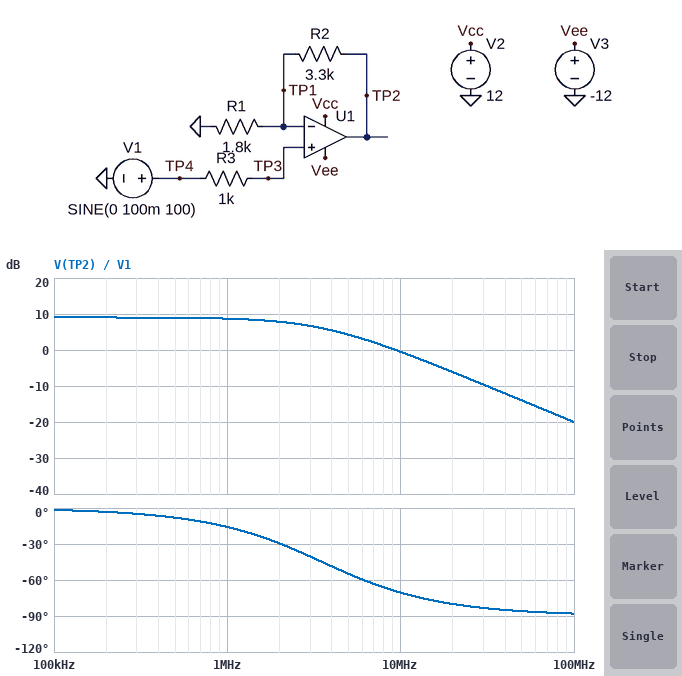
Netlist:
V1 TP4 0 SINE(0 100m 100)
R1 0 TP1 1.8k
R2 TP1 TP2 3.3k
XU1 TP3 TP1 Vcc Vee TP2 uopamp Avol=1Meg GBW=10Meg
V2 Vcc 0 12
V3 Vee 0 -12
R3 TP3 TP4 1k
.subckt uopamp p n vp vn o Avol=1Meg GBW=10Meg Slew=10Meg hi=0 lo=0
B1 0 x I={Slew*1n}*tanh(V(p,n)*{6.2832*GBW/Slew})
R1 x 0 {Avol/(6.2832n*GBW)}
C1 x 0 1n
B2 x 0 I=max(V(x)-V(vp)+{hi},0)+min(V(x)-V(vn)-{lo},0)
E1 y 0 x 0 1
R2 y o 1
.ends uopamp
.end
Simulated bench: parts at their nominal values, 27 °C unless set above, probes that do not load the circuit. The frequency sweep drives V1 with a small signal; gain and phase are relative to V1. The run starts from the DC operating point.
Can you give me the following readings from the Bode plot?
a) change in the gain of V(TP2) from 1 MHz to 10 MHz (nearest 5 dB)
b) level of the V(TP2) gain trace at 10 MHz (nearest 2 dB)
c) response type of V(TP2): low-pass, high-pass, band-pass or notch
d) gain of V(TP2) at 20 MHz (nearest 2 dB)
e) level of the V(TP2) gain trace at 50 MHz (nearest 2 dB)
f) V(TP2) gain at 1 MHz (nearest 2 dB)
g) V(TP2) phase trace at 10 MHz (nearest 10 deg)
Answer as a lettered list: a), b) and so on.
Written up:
a) -10 dB
b) 0 dB
c) low-pass
d) -6 dB
e) -14 dB
f) 8 dB
g) -70 deg
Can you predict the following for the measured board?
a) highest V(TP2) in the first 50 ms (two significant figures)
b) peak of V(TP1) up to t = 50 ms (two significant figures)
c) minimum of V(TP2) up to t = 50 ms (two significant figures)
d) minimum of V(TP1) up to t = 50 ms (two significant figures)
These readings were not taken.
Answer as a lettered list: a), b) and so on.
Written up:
a) 280 mV
b) 100 mV
c) -280 mV
d) -100 mV
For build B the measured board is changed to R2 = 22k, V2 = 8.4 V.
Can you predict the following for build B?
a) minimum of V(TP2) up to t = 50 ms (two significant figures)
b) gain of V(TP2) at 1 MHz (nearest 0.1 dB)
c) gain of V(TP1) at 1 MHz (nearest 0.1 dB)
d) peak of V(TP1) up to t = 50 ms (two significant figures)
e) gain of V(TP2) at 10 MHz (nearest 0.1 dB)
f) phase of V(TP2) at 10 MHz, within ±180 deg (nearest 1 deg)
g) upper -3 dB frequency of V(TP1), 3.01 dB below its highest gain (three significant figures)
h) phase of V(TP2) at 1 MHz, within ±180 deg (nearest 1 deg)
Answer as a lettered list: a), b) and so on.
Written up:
a) -1.3 V
b) 18.0 dB
c) -4.4 dB
d) 100 mV
e) 0 dB
f) -86 deg
g) 756 kHz
h) -53 deg
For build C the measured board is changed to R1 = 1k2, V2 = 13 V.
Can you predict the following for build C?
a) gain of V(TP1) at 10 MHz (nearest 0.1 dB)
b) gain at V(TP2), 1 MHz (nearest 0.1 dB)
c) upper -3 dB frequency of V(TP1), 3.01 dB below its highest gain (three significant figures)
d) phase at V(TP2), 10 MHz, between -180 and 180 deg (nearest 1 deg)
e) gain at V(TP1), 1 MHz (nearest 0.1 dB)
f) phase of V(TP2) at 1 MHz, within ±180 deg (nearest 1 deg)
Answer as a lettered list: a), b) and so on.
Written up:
a) -11.8 dB
b) 10.9 dB
c) 2.67 MHz
d) -75 deg
e) -0.6 dB
f) -21 deg
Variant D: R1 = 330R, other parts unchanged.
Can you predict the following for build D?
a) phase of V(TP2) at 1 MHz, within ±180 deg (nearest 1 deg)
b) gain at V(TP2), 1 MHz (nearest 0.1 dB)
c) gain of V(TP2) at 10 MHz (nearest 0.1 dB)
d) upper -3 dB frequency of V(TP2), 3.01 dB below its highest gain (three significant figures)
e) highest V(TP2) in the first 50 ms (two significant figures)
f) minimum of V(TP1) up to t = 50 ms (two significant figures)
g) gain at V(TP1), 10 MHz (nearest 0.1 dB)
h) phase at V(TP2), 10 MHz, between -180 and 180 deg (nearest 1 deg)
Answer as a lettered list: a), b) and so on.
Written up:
a) -48 deg
b) 17.4 dB
c) 0 dB
d) 909 kHz
e) 1.1 V
f) -100 mV
g) -20.9 dB
h) -85 deg
